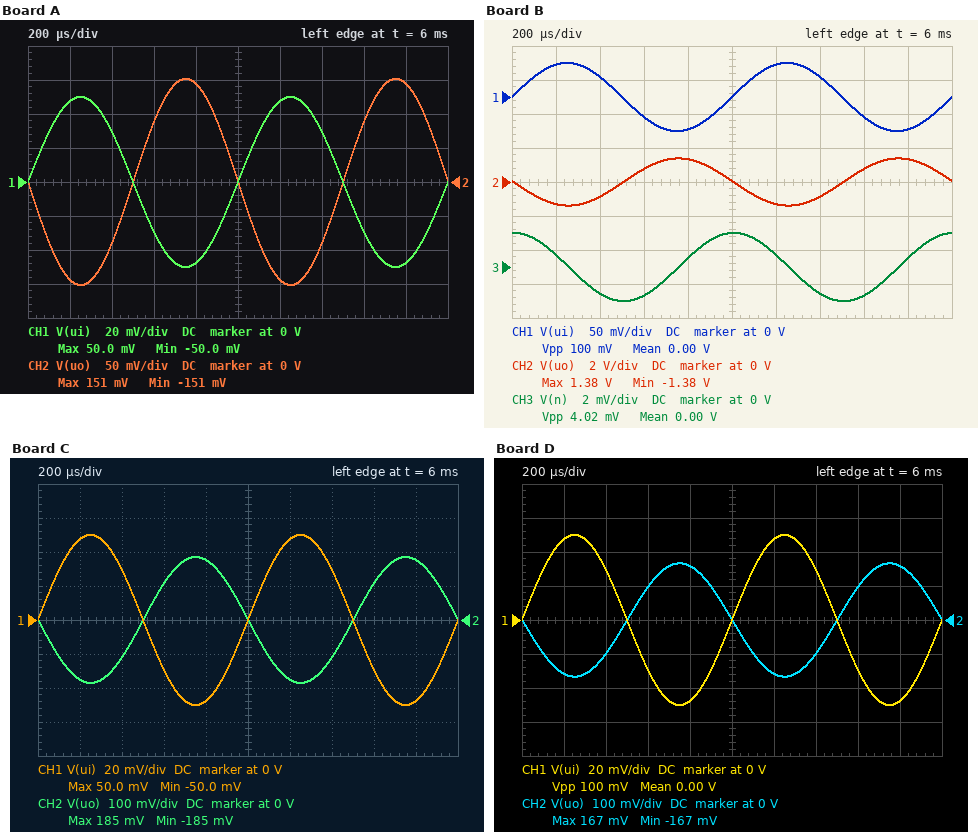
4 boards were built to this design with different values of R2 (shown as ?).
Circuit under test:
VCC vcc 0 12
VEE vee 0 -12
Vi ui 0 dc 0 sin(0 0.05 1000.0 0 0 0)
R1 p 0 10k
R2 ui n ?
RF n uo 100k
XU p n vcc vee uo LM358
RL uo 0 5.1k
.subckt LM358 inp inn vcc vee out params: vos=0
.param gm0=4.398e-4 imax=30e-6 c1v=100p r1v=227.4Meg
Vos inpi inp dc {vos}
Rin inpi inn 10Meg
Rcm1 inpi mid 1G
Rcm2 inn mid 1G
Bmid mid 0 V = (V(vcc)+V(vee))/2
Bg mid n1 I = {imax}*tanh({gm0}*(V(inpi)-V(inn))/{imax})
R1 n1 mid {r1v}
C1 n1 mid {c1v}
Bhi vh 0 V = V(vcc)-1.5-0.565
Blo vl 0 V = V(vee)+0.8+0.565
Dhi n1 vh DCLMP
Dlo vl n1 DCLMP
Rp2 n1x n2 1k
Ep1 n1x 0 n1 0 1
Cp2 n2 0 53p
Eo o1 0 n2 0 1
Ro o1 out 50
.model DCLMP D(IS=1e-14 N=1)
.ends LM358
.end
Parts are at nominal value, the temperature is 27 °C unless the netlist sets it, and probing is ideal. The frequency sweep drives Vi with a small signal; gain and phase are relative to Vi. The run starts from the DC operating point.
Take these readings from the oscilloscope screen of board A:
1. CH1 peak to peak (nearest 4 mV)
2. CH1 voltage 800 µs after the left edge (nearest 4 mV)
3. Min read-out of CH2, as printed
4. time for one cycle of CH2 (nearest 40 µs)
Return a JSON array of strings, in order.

["100 mV", "-48 mV", "-151 mV", "1.00 ms"]
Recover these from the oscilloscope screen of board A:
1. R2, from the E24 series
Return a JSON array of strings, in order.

["33 kΩ"]
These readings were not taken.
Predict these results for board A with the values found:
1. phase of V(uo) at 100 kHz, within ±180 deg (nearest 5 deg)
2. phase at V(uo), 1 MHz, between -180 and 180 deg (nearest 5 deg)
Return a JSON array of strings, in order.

["150 deg", "80 deg"]
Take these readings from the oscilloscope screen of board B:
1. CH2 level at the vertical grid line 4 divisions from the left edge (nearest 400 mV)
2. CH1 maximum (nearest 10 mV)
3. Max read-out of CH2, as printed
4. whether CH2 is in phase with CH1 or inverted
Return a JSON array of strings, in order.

["1.2 V", "50 mV", "1.38 V", "inverted"]
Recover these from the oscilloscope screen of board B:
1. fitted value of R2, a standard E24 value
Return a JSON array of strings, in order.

["3.6 kΩ"]
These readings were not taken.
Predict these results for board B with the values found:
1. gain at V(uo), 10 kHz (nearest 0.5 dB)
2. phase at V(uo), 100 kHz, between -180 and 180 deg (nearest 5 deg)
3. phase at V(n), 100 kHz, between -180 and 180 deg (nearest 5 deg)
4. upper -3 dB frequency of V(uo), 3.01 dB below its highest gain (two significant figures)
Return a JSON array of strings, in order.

["28.0 dB", "100 deg", "15 deg", "24 kHz"]
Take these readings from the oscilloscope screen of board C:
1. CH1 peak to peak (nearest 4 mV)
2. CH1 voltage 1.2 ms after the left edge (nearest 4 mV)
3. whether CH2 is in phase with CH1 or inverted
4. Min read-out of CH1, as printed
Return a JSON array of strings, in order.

["100 mV", "48 mV", "inverted", "-50.0 mV"]
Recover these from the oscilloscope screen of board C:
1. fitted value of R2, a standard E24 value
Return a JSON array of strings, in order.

["27 kΩ"]
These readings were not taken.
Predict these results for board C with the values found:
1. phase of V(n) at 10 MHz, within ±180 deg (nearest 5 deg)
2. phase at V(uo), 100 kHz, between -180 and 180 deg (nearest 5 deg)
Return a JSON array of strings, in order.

["0 deg", "145 deg"]
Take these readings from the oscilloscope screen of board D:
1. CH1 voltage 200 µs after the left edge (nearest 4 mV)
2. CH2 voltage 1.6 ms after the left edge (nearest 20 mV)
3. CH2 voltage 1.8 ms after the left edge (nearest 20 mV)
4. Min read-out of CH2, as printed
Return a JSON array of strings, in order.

["48 mV", "100 mV", "160 mV", "-167 mV"]
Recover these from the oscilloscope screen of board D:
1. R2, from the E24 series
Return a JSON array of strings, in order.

["30 kΩ"]
